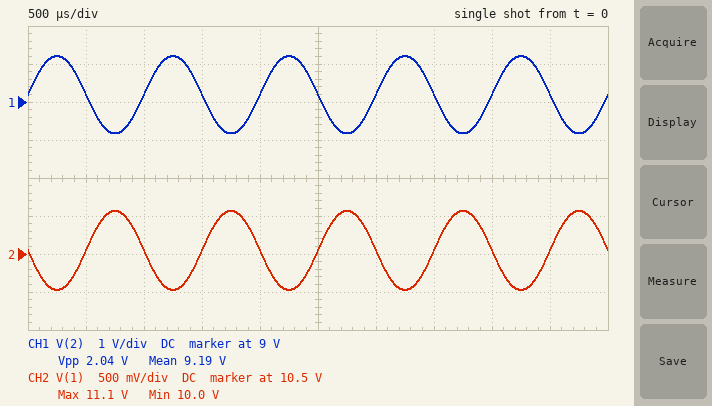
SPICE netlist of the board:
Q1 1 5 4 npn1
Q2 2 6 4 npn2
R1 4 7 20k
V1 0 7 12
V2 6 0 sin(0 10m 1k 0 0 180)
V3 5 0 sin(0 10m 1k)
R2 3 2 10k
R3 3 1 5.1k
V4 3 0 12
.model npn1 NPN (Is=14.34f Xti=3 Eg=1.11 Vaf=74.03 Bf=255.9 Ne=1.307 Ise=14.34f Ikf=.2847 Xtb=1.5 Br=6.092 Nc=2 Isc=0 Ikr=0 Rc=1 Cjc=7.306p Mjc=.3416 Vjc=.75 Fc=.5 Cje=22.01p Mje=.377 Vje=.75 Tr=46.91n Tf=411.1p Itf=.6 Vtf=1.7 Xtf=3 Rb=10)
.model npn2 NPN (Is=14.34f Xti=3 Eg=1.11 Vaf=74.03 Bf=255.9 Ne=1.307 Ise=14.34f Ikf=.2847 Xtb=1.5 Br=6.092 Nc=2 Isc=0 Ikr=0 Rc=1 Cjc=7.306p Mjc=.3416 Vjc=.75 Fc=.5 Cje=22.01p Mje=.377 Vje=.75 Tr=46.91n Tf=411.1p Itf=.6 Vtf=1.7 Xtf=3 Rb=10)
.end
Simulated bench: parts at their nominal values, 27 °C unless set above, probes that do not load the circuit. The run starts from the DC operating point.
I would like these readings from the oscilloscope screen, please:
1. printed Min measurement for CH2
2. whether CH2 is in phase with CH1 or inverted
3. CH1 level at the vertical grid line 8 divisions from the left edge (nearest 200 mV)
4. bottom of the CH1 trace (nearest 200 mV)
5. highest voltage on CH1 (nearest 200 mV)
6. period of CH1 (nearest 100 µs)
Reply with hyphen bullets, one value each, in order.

- 10.0 V
- inverted
- 9.2 V
- 8.2 V
- 10.2 V
- 1.0 ms
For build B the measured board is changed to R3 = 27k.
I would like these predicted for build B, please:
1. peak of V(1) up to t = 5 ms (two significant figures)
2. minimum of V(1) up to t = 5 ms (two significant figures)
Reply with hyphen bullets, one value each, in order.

- 7.2 V
- 1.9 V
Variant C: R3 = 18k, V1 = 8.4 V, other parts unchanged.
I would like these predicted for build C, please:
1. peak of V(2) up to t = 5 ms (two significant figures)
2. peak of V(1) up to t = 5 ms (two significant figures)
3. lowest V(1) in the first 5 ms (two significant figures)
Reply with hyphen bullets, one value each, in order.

- 11 V
- 9.8 V
- 7.3 V
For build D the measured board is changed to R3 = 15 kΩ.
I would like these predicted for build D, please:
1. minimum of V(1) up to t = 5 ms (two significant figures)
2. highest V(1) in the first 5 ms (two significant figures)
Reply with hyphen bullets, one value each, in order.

- 6.3 V
- 9.3 V
